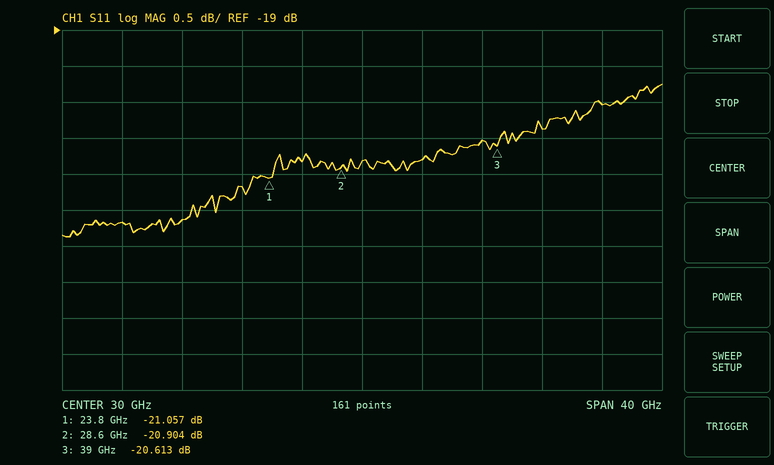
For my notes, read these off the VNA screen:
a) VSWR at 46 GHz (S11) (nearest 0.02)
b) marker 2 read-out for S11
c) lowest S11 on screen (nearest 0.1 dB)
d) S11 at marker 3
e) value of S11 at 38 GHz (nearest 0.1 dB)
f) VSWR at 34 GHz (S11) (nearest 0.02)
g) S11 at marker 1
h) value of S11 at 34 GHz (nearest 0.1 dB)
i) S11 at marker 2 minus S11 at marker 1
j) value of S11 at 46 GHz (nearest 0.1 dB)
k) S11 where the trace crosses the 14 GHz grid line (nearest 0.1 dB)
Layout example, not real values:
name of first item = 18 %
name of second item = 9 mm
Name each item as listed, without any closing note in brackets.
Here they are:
VSWR at 46 GHz (S11) = 1.22
marker 2 read-out for S11 = -20.904 dB
lowest S11 on screen = -21.9 dB
S11 at marker 3 = -20.613 dB
value of S11 at 38 GHz = -20.5 dB
VSWR at 34 GHz (S11) = 1.20
S11 at marker 1 = -21.057 dB
value of S11 at 34 GHz = -20.8 dB
S11 at marker 2 minus S11 at marker 1 = 0.153 dB
value of S11 at 46 GHz = -20.0 dB
S11 where the trace crosses the 14 GHz grid line = -21.7 dB
